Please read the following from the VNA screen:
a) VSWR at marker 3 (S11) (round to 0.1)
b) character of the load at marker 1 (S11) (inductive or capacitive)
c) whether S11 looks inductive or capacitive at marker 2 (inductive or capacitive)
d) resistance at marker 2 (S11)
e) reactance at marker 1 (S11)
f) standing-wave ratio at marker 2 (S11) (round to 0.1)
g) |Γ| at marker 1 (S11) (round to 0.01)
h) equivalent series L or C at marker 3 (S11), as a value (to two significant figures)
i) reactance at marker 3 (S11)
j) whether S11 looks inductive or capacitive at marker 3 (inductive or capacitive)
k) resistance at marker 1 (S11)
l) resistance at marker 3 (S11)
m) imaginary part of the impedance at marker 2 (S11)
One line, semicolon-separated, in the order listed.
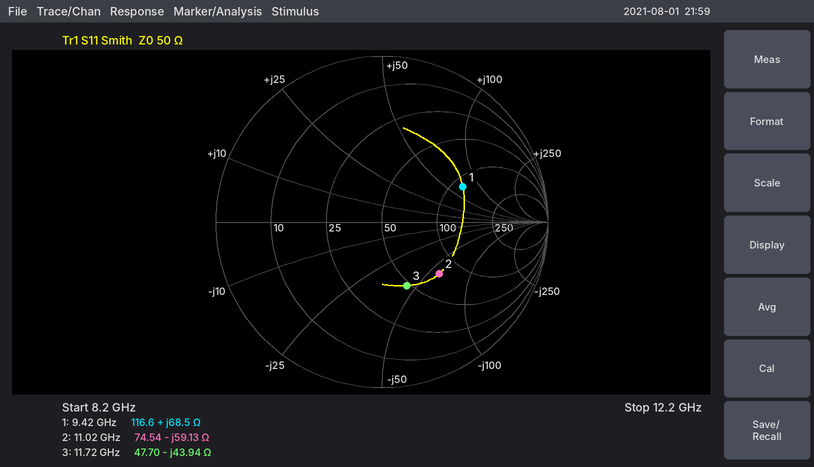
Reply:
2.4; inductive; capacitive; 74.54 Ω; +68.5 Ω; 2.7; 0.53; 310 fF; -43.94 Ω; capacitive; 116.6 Ω; 47.70 Ω; -59.13 Ω
